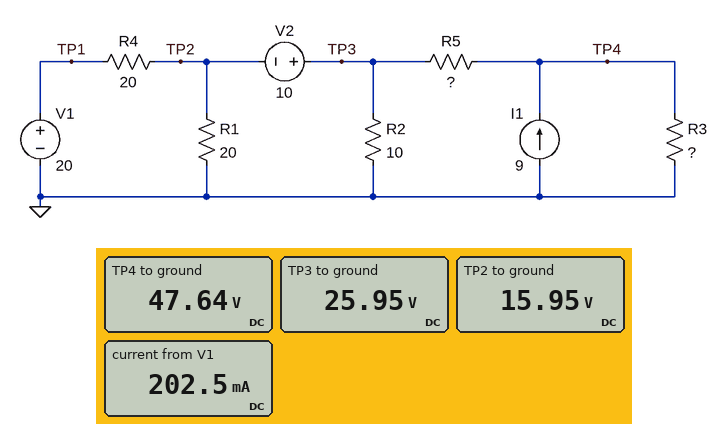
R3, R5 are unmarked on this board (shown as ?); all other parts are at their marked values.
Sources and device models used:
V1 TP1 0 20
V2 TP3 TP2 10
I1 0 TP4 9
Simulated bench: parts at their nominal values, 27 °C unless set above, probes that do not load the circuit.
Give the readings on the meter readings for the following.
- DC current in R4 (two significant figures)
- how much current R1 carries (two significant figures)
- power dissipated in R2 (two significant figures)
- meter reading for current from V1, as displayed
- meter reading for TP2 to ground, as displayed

200 mA
800 mA
67 W
202.5 mA
15.95 V
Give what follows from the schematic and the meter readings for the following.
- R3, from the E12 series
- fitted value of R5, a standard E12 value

8.2 Ω
6.8 Ω
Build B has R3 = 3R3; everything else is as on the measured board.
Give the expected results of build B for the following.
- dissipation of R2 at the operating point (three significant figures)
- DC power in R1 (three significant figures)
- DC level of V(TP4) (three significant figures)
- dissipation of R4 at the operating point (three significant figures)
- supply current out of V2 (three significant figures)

27.3 W
2.13 W
25.4 V
9.08 W
348 mA
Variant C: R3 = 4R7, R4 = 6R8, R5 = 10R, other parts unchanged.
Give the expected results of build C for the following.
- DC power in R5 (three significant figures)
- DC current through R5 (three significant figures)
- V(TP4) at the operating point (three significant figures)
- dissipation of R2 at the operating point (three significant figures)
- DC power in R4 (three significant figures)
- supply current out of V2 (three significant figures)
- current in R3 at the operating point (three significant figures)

20.3 W
1.43 A
35.6 V
45.5 W
11.0 W
707 mA
7.57 A
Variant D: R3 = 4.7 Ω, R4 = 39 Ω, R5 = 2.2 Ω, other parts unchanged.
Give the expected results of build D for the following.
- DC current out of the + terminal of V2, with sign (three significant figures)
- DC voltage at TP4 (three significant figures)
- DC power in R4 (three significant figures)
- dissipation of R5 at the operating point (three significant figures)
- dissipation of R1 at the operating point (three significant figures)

-477 mA
29.2 V
1.23 W
17.1 W
8.56 W
